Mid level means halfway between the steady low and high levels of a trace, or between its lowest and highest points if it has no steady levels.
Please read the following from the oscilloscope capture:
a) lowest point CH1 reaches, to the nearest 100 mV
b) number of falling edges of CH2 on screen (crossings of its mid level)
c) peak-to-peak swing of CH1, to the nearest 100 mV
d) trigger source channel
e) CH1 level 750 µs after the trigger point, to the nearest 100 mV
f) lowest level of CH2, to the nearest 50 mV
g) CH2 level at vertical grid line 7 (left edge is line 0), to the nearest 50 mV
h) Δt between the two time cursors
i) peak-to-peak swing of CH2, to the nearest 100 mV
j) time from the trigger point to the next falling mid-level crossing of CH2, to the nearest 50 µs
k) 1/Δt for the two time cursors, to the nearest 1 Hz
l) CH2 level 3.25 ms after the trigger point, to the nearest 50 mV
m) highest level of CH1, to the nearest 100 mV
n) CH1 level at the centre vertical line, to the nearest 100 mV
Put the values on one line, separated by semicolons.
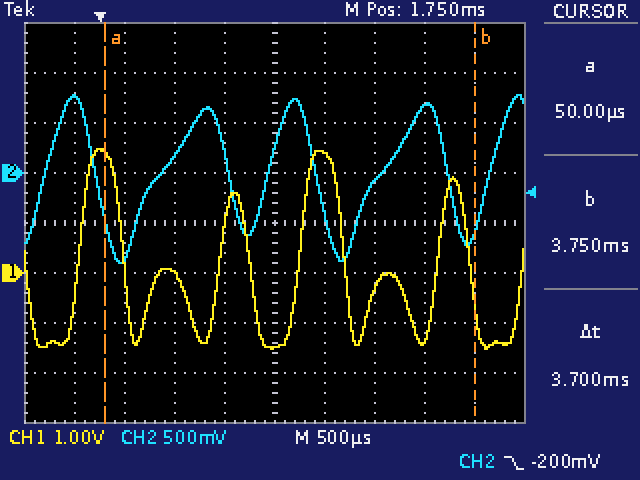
-1.5 V; 4; 4.0 V; CH2; 0.0 V; -900 mV; -100 mV; 3.7 ms; 1.70 V; 1.30 ms; 270 Hz; 650 mV; 2.5 V; -1.5 V
